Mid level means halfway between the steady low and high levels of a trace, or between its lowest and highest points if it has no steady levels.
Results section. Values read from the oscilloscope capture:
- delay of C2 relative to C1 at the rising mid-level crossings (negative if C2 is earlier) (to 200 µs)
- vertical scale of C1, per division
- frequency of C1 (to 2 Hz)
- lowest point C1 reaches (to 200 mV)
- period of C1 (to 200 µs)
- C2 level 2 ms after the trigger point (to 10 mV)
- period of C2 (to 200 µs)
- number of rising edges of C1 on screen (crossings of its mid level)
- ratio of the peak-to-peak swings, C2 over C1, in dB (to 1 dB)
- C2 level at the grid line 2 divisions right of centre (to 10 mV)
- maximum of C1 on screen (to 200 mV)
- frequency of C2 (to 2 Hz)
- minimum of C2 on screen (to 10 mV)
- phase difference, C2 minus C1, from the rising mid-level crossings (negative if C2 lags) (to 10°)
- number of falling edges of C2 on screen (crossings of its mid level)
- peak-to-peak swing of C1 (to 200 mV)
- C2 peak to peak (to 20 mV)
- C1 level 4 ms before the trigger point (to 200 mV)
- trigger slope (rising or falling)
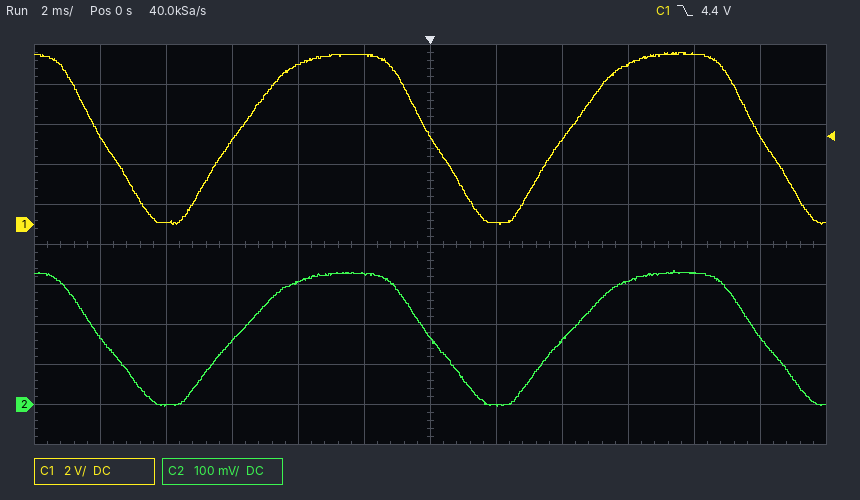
0.0 ms
2 V
100 Hz
0.0 V
10.0 ms
0 mV
10.0 ms
2
-28 dB
160 mV
8.6 V
100 Hz
0 mV
0°
3
8.6 V
340 mV
8.0 V
falling
